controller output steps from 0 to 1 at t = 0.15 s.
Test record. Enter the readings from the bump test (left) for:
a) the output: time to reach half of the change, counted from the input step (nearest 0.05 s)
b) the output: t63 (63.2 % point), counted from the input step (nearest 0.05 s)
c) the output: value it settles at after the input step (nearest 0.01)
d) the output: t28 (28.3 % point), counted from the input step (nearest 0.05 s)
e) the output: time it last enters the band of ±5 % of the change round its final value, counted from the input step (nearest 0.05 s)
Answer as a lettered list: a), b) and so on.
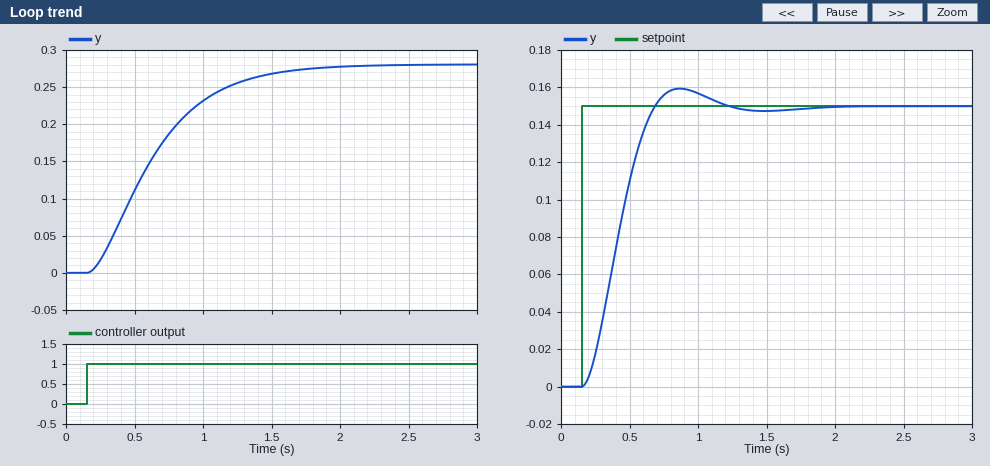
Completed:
a) 0.45 s
b) 0.55 s
c) 0.28
d) 0.25 s
e) 1.30 s
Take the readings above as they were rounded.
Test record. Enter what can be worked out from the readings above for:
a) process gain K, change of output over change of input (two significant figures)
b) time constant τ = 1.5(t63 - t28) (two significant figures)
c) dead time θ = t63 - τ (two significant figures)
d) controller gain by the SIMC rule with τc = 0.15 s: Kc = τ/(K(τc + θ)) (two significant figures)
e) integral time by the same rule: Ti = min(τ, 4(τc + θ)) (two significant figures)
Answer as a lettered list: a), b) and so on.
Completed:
a) 0.28
b) 0.45 s
c) 0.10 s
d) 6.4
e) 0.45 s
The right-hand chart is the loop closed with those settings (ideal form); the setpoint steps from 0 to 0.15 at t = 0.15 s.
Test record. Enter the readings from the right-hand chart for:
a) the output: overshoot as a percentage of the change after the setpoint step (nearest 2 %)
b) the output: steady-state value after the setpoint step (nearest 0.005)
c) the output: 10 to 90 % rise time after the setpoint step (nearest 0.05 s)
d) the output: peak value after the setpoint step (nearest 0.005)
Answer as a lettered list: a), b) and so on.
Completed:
a) 6 %
b) 0.150
c) 0.35 s
d) 0.160
